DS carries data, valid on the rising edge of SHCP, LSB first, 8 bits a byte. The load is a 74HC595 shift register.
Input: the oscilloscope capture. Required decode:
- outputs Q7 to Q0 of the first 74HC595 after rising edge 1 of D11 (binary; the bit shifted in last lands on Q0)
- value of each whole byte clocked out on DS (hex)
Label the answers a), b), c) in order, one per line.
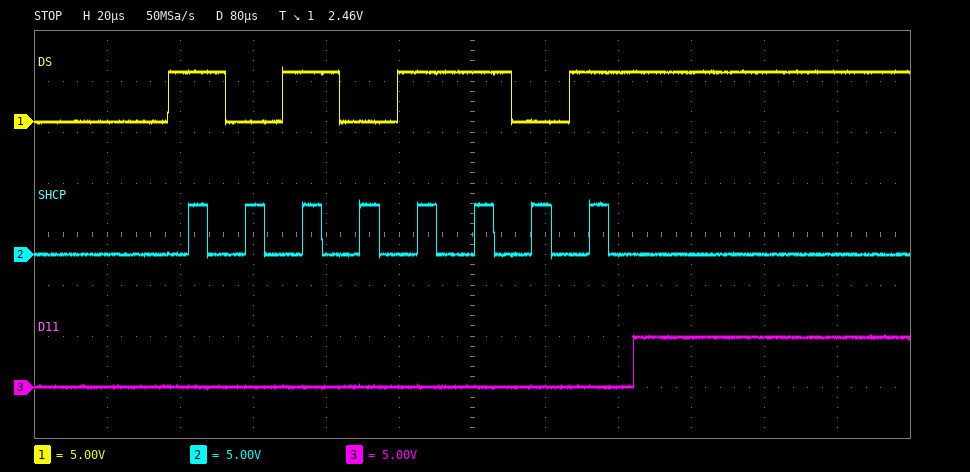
a) 10101101
b) B5
